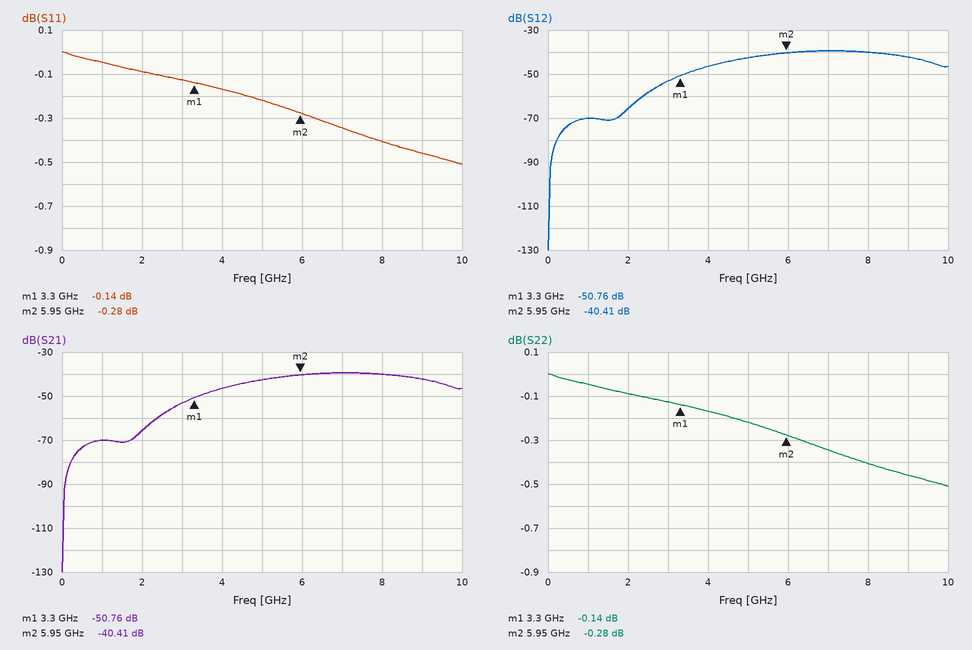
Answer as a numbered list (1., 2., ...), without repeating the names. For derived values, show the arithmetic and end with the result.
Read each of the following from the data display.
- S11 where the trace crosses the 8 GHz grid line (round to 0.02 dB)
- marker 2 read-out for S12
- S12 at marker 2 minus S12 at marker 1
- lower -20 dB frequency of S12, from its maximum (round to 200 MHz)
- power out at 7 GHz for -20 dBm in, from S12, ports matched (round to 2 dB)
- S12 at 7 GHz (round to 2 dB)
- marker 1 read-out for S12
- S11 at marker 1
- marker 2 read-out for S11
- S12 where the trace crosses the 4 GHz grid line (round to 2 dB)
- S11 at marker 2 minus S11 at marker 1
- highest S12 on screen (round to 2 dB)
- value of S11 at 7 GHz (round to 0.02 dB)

1. -0.40 dB
2. -40.41 dB
3. -40.41 − (-50.76) = 10.35 dB
4. 2.4 GHz
5. -20 dBm + (-40 dB) = -60 dBm
6. -40 dB
7. -50.76 dB
8. -0.14 dB
9. -0.28 dB
10. -46 dB
11. -0.28 − (-0.14) = -0.14 dB
12. -40 dB
13. -0.34 dB
